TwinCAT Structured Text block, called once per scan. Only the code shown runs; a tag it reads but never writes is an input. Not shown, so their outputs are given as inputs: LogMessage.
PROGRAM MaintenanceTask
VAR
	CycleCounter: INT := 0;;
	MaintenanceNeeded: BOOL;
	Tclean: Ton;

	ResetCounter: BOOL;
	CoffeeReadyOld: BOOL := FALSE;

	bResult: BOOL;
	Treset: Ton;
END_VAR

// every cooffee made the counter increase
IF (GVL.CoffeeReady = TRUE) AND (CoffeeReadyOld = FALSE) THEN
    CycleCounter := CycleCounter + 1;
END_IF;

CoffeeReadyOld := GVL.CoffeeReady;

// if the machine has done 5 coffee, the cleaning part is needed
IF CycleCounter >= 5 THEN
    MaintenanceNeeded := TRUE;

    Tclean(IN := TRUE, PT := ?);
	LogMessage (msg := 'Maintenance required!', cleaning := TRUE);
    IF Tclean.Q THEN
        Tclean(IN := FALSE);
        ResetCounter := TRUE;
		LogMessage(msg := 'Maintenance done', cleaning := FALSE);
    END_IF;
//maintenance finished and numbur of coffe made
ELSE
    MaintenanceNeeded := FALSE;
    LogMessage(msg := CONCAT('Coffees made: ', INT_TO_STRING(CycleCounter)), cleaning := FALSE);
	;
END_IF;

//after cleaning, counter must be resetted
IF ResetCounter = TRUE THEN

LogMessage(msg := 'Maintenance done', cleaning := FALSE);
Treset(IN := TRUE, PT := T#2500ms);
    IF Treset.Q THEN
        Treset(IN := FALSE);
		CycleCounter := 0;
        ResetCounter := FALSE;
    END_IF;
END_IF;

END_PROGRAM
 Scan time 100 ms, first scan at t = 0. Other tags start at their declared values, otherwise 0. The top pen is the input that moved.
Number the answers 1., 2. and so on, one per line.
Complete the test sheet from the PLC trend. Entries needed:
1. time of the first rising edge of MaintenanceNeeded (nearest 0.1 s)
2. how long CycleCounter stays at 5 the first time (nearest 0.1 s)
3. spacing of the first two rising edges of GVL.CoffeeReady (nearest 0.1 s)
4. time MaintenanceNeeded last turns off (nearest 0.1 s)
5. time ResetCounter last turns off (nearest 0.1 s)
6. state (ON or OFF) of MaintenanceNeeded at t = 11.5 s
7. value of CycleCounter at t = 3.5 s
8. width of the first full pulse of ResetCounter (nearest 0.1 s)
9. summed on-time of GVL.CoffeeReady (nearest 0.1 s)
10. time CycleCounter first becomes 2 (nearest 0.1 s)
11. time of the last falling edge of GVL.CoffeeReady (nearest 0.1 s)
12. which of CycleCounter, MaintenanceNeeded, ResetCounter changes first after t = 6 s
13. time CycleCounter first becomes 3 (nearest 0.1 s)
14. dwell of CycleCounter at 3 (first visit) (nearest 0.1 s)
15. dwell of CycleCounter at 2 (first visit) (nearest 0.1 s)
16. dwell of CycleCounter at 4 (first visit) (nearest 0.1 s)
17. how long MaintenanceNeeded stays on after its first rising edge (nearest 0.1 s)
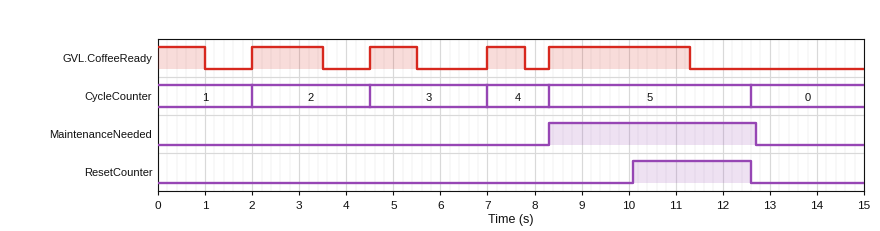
1. 8.3 s
2. 4.3 s
3. 2.5 s
4. 12.7 s
5. 12.6 s
6. ON
7. 2
8. 2.5 s
9. 7.3 s
10. 2.0 s
11. 11.3 s
12. CycleCounter
13. 4.5 s
14. 2.5 s
15. 2.5 s
16. 1.3 s
17. 4.4 s
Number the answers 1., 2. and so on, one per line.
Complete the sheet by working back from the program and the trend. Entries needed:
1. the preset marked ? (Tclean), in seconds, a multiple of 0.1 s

1. 1.8 s
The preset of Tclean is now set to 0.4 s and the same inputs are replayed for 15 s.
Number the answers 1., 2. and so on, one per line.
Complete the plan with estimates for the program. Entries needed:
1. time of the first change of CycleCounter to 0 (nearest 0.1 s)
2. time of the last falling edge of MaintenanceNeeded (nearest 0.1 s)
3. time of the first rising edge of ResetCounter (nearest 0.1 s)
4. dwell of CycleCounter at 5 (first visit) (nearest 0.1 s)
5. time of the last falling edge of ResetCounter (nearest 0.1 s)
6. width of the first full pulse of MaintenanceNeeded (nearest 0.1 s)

1. 11.2 s
2. 11.3 s
3. 8.7 s
4. 2.9 s
5. 11.2 s
6. 3.0 s
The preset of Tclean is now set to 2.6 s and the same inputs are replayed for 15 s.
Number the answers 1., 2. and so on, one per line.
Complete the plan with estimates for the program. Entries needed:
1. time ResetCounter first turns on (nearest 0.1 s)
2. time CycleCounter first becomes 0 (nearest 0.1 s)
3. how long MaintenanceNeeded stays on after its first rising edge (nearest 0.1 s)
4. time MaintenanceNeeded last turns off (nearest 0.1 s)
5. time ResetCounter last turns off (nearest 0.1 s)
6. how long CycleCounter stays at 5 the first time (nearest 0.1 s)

1. 10.9 s
2. 13.4 s
3. 5.2 s
4. 13.5 s
5. 13.4 s
6. 5.1 s
